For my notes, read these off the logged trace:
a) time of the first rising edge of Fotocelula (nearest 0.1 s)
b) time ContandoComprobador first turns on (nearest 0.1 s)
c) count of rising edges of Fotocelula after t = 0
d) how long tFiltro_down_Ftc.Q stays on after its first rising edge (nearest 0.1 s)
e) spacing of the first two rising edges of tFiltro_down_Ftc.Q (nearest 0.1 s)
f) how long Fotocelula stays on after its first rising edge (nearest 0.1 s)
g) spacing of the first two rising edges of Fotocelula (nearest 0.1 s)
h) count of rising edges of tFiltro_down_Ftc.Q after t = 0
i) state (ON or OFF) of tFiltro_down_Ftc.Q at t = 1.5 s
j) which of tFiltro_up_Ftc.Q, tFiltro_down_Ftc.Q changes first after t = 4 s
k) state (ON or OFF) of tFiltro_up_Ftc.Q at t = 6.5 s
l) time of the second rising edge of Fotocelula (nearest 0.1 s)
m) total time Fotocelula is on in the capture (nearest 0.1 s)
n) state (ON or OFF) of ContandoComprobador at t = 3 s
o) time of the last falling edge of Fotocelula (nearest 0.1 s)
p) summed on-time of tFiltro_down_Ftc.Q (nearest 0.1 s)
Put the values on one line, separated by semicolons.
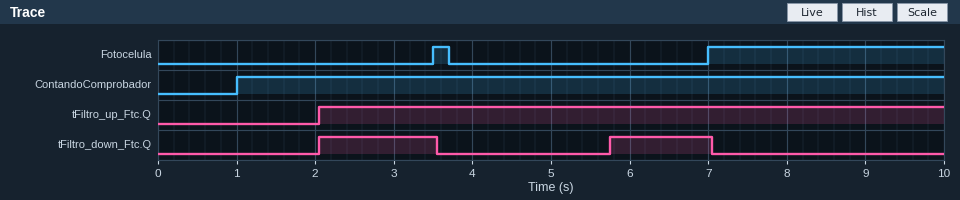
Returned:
3.5 s; 1.0 s; 2; 1.5 s; 3.7 s; 0.2 s; 3.5 s; 2; OFF; tFiltro_down_Ftc.Q; ON; 7.0 s; 3.2 s; ON; 3.7 s; 2.8 s
